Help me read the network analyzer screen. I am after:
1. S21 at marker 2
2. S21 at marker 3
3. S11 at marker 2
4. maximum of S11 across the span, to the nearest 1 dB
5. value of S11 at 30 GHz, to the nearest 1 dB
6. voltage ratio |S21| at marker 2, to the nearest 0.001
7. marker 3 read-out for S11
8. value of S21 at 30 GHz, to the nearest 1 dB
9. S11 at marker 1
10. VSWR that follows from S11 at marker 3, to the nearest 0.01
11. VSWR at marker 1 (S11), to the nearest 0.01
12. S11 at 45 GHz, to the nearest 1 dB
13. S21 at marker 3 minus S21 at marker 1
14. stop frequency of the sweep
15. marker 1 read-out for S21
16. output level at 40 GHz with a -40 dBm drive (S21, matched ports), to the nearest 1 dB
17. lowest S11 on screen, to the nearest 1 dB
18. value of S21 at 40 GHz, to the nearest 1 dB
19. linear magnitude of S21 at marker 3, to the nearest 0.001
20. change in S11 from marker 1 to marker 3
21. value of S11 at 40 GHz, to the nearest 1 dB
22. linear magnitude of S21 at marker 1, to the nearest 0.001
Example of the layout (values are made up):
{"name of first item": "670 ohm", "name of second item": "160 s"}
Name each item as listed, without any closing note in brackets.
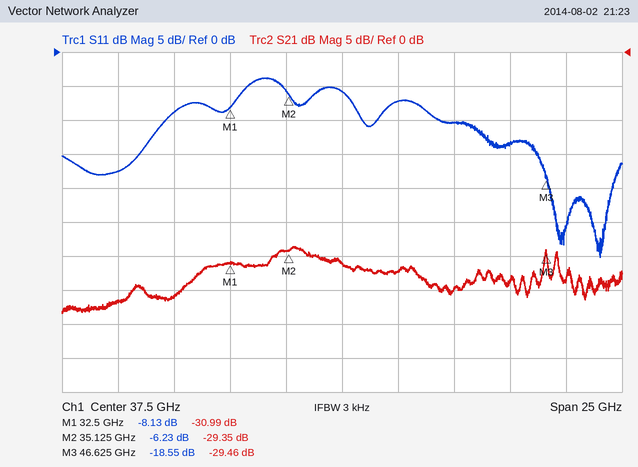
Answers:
{"S21 at marker 2": "-29.35 dB", "S21 at marker 3": "-29.46 dB", "S11 at marker 2": "-6.23 dB", "maximum of S11 across the span, to the nearest 1 dB": "-4 dB", "value of S11 at 30 GHz, to the nearest 1 dB": "-9 dB", "voltage ratio |S21| at marker 2, to the nearest 0.001": "0.034", "marker 3 read-out for S11": "-18.55 dB", "value of S21 at 30 GHz, to the nearest 1 dB": "-36 dB", "S11 at marker 1": "-8.13 dB", "VSWR that follows from S11 at marker 3, to the nearest 0.01": "1.27", "VSWR at marker 1 (S11), to the nearest 0.01": "2.29", "S11 at 45 GHz, to the nearest 1 dB": "-13 dB", "S21 at marker 3 minus S21 at marker 1": "1.53 dB", "stop frequency of the sweep": "50 GHz", "marker 1 read-out for S21": "-30.99 dB", "output level at 40 GHz with a -40 dBm drive (S21, matched ports), to the nearest 1 dB": "-72 dBm", "lowest S11 on screen, to the nearest 1 dB": "-30 dB", "value of S21 at 40 GHz, to the nearest 1 dB": "-32 dB", "linear magnitude of S21 at marker 3, to the nearest 0.001": "0.034", "change in S11 from marker 1 to marker 3": "-10.42 dB", "value of S11 at 40 GHz, to the nearest 1 dB": "-7 dB", "linear magnitude of S21 at marker 1, to the nearest 0.001": "0.028"}
